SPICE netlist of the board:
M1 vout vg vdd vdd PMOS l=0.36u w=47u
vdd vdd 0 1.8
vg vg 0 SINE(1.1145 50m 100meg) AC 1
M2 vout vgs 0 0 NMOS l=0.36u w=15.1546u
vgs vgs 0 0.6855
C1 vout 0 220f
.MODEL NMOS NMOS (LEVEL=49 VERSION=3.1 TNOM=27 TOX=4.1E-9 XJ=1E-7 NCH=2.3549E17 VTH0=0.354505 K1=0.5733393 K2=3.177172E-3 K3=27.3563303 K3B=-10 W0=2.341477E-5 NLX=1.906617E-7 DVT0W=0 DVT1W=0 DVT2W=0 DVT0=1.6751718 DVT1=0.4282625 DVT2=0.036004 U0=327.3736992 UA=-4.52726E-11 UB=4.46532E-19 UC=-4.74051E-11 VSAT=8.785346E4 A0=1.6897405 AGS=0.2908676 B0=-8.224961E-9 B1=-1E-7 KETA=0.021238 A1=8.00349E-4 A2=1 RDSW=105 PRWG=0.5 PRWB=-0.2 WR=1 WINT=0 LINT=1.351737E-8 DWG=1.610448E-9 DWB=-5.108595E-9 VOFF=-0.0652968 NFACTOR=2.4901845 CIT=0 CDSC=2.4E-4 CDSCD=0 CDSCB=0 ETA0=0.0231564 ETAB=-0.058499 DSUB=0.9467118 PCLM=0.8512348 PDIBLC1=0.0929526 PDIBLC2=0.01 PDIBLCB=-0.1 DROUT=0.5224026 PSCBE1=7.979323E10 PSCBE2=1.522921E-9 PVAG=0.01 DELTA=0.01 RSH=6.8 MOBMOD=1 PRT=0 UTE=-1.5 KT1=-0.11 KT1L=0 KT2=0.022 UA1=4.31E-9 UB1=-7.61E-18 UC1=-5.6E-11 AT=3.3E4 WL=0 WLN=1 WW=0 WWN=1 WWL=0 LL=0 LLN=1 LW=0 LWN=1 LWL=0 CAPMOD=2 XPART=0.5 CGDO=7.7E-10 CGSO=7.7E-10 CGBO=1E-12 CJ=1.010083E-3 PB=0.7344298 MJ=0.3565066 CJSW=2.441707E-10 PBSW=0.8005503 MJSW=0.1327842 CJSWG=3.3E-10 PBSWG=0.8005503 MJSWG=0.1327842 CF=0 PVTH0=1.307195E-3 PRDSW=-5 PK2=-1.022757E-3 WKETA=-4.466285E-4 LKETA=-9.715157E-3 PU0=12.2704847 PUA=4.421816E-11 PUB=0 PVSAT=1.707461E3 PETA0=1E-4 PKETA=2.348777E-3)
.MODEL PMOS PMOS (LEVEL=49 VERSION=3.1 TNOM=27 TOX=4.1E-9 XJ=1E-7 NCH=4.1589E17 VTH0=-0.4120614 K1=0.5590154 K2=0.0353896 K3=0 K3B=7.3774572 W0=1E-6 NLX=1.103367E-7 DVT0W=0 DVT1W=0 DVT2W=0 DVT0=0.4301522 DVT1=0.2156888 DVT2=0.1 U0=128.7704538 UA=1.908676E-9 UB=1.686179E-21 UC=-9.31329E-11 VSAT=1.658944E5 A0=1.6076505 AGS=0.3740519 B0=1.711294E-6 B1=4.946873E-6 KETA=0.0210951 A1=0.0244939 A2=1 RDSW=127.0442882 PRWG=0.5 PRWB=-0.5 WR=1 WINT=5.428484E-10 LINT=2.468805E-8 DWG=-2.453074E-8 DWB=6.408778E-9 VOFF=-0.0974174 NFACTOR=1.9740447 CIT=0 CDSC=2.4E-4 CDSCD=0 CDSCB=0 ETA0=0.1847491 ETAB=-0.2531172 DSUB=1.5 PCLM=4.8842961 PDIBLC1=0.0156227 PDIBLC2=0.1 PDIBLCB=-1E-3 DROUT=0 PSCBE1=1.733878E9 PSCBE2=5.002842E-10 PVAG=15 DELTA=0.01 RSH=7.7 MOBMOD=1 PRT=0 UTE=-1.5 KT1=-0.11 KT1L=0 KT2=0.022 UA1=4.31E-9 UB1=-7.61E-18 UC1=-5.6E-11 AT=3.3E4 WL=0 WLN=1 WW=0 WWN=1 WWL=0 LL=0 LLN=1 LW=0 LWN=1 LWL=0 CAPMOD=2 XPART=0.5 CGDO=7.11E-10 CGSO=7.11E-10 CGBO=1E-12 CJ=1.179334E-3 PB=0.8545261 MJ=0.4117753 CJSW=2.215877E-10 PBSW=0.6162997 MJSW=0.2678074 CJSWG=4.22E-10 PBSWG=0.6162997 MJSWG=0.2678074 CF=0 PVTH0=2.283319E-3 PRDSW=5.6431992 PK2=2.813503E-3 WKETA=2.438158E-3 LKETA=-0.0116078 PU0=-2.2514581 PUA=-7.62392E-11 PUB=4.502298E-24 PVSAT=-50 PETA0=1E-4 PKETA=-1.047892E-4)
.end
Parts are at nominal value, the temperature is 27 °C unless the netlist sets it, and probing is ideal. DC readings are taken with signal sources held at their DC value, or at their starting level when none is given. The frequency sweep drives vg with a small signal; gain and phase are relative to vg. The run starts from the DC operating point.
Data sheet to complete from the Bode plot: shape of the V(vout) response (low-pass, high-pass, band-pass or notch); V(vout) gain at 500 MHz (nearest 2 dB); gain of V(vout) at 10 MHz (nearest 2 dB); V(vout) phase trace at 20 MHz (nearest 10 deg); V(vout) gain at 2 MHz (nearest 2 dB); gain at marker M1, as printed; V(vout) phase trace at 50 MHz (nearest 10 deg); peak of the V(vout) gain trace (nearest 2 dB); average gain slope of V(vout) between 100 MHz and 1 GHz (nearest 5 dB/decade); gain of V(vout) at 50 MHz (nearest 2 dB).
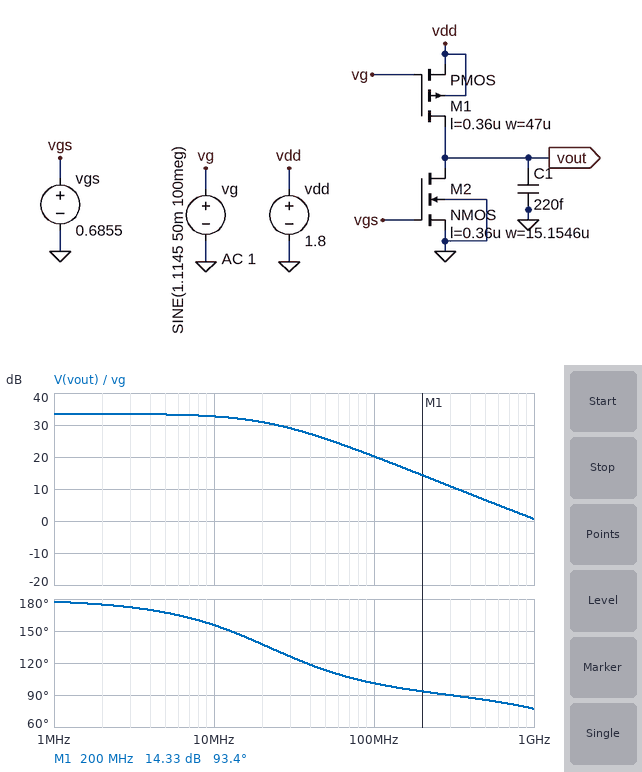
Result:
low-pass
6 dB
32 dB
140 deg
34 dB
14.33 dB
110 deg
34 dB
-20 dB/decade
26 dB
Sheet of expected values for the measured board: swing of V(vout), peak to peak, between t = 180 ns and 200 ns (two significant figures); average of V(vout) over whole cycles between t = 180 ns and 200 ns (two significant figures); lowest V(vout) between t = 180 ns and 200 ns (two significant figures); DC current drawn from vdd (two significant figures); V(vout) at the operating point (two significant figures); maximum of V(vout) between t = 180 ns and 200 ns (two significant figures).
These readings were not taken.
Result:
1.0 V
990 mV
490 mV
220 µA
880 mV
1.5 V
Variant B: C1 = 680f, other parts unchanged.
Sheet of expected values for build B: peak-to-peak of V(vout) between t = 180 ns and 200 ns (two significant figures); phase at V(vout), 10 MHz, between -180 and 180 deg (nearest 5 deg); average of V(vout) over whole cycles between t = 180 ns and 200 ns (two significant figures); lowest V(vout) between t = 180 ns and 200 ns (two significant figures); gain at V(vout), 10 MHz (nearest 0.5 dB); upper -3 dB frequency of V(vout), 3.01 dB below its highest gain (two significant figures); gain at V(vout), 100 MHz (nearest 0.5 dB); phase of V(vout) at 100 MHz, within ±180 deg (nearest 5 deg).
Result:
390 mV
130 deg
1.0 V
800 mV
29.5 dB
8.5 MHz
12.0 dB
95 deg
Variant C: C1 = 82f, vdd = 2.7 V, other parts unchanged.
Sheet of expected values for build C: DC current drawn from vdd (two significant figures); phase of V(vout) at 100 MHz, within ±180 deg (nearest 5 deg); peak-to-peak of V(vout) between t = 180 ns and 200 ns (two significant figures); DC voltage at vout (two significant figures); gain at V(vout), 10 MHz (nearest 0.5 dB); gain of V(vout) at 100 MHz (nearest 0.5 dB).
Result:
250 µA
155 deg
2.1 mV
2.7 V
-34.5 dB
-33.5 dB
